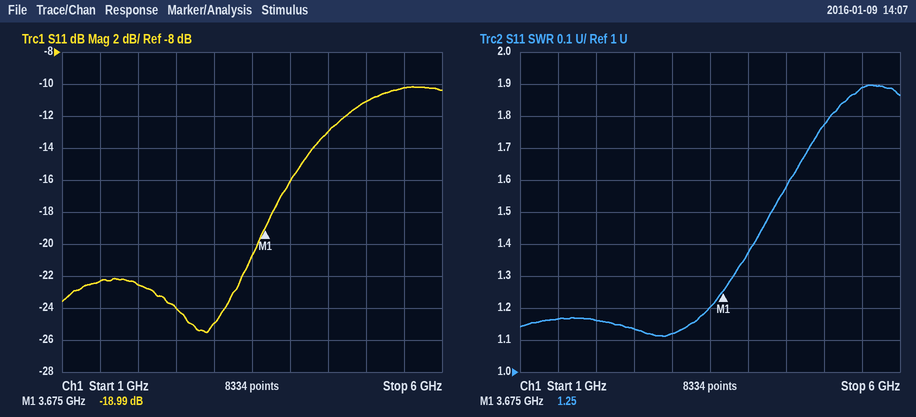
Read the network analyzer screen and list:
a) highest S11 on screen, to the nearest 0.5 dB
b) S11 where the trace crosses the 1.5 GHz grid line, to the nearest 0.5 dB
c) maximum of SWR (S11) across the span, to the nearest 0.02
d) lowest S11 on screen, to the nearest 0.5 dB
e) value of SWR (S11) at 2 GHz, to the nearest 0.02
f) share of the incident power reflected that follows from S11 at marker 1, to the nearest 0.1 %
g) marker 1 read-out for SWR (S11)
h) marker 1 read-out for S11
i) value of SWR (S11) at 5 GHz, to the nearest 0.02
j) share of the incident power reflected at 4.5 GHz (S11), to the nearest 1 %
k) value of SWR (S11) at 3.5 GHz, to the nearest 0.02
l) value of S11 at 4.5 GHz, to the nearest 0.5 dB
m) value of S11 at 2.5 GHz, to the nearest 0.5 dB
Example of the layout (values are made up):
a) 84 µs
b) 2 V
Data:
a) -10.0 dB
b) -22.5 dB
c) 1.90
d) -25.5 dB
e) 1.16
f) 1.3 %
g) 1.25
h) -18.99 dB
i) 1.78
j) 5 %
k) 1.20
l) -13.0 dB
m) -24.0 dB
